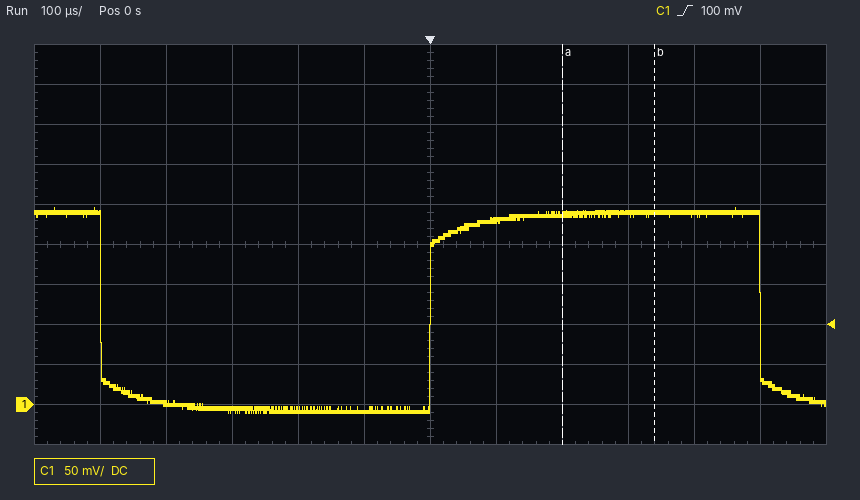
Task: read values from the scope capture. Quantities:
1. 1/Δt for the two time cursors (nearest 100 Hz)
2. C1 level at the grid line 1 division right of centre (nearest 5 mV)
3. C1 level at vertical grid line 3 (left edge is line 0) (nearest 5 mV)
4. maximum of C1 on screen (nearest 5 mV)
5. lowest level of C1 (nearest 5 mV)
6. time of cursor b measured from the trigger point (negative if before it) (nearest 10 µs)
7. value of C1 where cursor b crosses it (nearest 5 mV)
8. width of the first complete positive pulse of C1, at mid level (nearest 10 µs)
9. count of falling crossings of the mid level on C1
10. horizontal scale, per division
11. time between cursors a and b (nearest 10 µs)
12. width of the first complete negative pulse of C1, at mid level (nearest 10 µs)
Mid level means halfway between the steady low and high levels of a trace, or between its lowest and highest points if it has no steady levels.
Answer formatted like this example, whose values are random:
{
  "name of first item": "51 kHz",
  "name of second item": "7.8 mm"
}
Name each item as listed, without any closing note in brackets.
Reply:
{
  "1/Δt for the two time cursors": "7.1 kHz",
  "C1 level at the grid line 1 division right of centre": "230 mV",
  "C1 level at vertical grid line 3 (left edge is line 0)": "-5 mV",
  "maximum of C1 on screen": "245 mV",
  "lowest level of C1": "-10 mV",
  "time of cursor b measured from the trigger point (negative if before it)": "+340 µs",
  "value of C1 where cursor b crosses it": "240 mV",
  "width of the first complete positive pulse of C1, at mid level": "500 µs",
  "count of falling crossings of the mid level on C1": "2",
  "horizontal scale, per division": "100 µs",
  "time between cursors a and b": "140 µs",
  "width of the first complete negative pulse of C1, at mid level": "500 µs"
}
